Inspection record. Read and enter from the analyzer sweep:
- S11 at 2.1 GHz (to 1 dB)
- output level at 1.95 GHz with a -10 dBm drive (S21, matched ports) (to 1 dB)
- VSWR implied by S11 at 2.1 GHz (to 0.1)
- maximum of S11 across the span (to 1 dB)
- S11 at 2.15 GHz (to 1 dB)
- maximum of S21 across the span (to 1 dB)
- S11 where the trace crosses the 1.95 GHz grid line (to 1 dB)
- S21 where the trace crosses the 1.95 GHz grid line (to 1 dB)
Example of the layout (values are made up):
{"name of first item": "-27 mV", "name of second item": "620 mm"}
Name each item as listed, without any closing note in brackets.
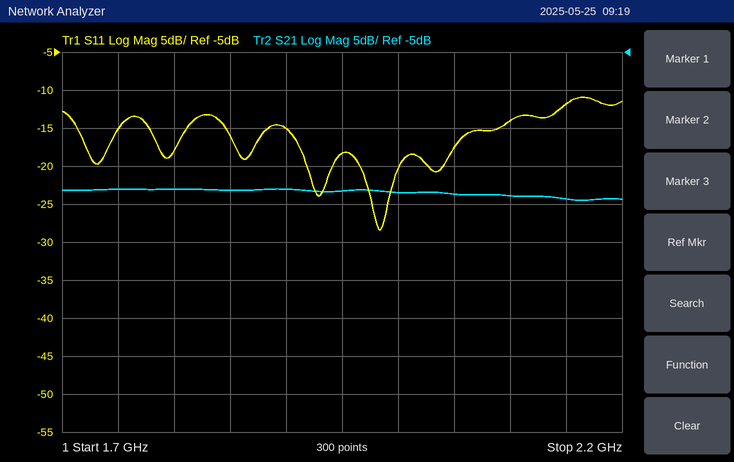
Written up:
{"S11 at 2.1 GHz": "-14 dB", "output level at 1.95 GHz with a -10 dBm drive (S21, matched ports)": "-33 dBm", "VSWR implied by S11 at 2.1 GHz": "1.5", "maximum of S11 across the span": "-11 dB", "S11 at 2.15 GHz": "-12 dB", "maximum of S21 across the span": "-23 dB", "S11 where the trace crosses the 1.95 GHz grid line": "-18 dB", "S21 where the trace crosses the 1.95 GHz grid line": "-23 dB"}
